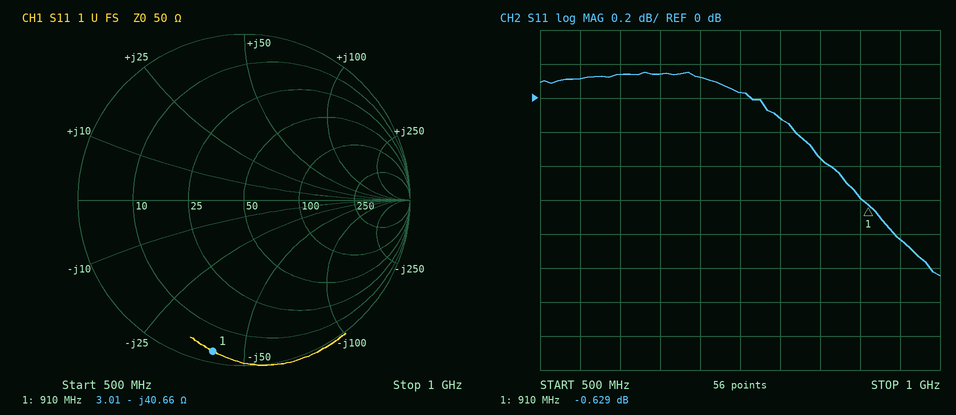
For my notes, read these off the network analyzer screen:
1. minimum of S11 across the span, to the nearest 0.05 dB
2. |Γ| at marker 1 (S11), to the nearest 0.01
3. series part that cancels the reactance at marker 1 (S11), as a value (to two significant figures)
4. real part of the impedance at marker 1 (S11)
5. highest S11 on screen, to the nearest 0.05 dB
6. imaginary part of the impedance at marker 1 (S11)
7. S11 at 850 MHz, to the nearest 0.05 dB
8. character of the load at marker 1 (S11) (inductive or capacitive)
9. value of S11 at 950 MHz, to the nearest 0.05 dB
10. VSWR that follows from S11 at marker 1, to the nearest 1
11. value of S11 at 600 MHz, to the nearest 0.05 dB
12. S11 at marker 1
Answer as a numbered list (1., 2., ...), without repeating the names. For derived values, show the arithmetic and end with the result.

1. -1.05 dB
2. 0.93
3. L = 40.66 Ω/(2π × 910 MHz) ≈ 7.1 nH
4. 3.01 Ω
5. 0.15 dB
6. -40.66 Ω
7. -0.35 dB
8. capacitive
9. -0.85 dB
10. (1 + 0.9301)/(1 − 0.9301) ≈ 28
11. 0.15 dB
12. -0.629 dB
